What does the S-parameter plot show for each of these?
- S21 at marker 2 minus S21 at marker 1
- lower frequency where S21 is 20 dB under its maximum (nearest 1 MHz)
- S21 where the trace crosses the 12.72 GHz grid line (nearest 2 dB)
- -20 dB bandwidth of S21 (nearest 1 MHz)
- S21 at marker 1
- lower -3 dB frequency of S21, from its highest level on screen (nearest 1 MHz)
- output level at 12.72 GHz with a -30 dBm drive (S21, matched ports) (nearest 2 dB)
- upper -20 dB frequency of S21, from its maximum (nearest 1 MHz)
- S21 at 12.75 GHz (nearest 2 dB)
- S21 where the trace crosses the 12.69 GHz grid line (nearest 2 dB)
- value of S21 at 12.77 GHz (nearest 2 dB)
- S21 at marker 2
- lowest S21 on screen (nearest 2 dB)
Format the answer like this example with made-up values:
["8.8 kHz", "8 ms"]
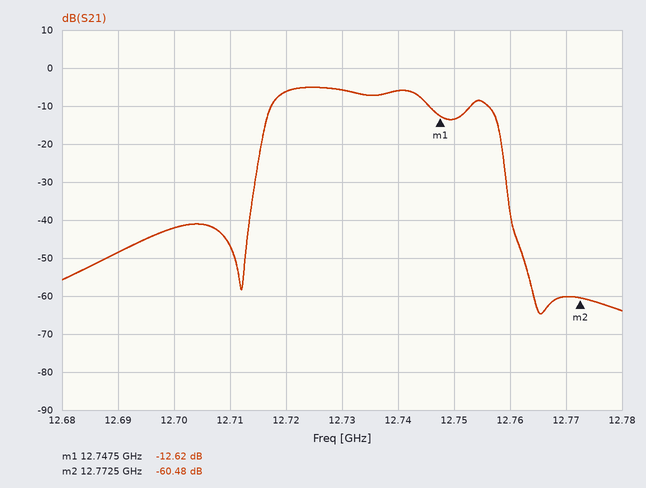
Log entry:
["-47.86 dB", "12.715 GHz", "-6 dB", "44 MHz", "-12.62 dB", "12.718 GHz", "-36 dBm", "12.759 GHz", "-14 dB", "-48 dB", "-60 dB", "-60.48 dB", "-64 dB"]
